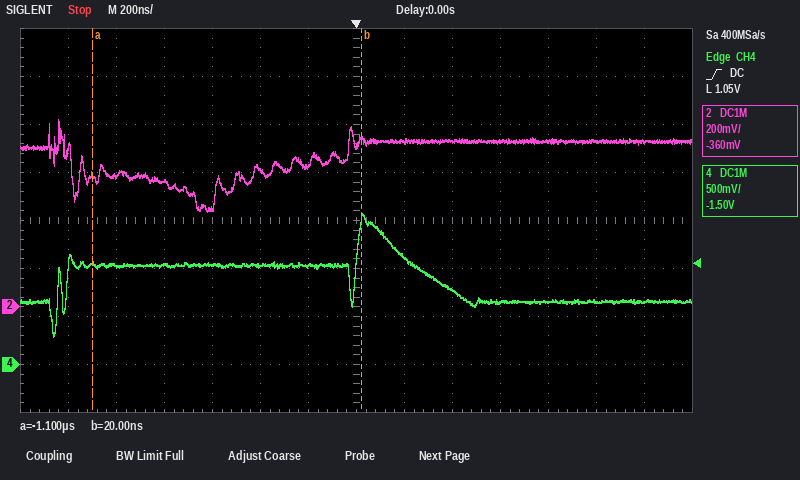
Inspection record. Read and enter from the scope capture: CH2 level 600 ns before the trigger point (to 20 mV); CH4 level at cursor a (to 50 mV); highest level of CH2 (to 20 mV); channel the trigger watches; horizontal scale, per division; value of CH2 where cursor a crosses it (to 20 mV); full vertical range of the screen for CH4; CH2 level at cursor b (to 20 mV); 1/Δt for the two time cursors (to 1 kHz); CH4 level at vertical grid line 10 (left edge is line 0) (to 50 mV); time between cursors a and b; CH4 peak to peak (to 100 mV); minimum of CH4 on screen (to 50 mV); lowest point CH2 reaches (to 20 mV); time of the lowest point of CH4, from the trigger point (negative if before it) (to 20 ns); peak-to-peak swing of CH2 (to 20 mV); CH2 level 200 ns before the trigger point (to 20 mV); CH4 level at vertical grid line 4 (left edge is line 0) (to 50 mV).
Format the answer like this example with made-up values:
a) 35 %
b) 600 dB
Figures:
a) 420 mV
b) 1.05 V
c) 780 mV
d) CH4
e) 200 ns
f) 540 mV
g) 4 V
h) 700 mV
i) 893 kHz
j) 650 mV
k) 1.12 µs
l) 1.30 V
m) 300 mV
n) 400 mV
o) -1.26 µs
p) 380 mV
q) 580 mV
r) 1.05 V
